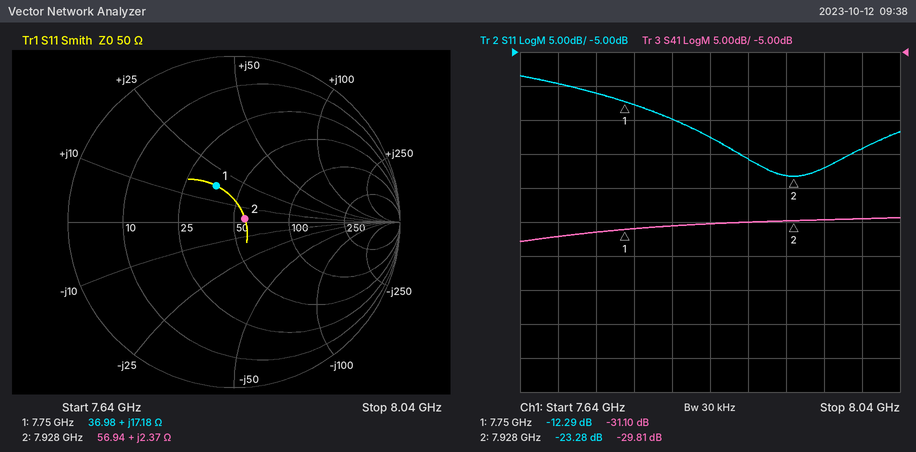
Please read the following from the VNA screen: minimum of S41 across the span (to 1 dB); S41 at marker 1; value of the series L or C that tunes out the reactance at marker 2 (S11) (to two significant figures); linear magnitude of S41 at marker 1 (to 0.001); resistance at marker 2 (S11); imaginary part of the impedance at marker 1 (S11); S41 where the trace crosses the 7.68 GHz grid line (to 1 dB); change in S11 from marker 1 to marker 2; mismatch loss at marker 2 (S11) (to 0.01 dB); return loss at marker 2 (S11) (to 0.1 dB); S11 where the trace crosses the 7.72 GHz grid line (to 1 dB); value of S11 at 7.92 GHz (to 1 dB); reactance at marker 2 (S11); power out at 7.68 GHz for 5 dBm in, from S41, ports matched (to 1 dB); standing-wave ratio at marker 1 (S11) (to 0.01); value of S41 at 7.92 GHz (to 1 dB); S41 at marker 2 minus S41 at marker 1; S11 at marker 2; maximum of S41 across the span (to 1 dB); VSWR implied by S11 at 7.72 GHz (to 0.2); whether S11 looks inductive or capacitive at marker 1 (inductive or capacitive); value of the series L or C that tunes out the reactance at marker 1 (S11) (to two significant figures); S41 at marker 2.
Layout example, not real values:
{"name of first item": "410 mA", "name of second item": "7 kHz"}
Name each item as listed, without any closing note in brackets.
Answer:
{"minimum of S41 across the span": "-33 dB", "S41 at marker 1": "-31.10 dB", "value of the series L or C that tunes out the reactance at marker 2 (S11)": "8.5 pF", "linear magnitude of S41 at marker 1": "0.028", "resistance at marker 2": "56.94 Ω", "imaginary part of the impedance at marker 1": "+17.18 Ω", "S41 where the trace crosses the 7.68 GHz grid line": "-32 dB", "change in S11 from marker 1 to marker 2": "-10.99 dB", "mismatch loss at marker 2 (S11)": "0.02 dB", "return loss at marker 2 (S11)": "23.3 dB", "S11 where the trace crosses the 7.72 GHz grid line": "-11 dB", "value of S11 at 7.92 GHz": "-23 dB", "reactance at marker 2": "+2.37 Ω", "power out at 7.68 GHz for 5 dBm in, from S41, ports matched": "-27 dBm", "standing-wave ratio at marker 1 (S11)": "1.64", "value of S41 at 7.92 GHz": "-30 dB", "S41 at marker 2 minus S41 at marker 1": "1.29 dB", "S11 at marker 2": "-23.28 dB", "maximum of S41 across the span": "-29 dB", "VSWR implied by S11 at 7.72 GHz": "1.8", "whether S11 looks inductive or capacitive at marker 1": "inductive", "value of the series L or C that tunes out the reactance at marker 1 (S11)": "1.2 pF", "S41 at marker 2": "-29.81 dB"}
